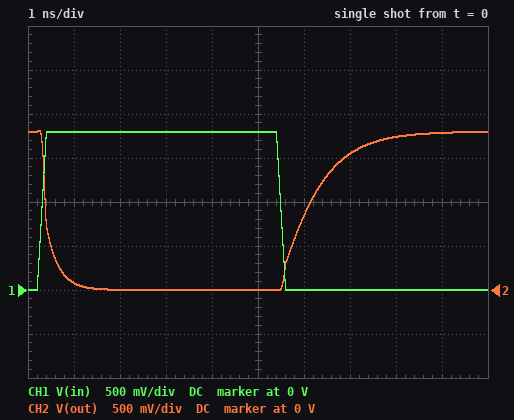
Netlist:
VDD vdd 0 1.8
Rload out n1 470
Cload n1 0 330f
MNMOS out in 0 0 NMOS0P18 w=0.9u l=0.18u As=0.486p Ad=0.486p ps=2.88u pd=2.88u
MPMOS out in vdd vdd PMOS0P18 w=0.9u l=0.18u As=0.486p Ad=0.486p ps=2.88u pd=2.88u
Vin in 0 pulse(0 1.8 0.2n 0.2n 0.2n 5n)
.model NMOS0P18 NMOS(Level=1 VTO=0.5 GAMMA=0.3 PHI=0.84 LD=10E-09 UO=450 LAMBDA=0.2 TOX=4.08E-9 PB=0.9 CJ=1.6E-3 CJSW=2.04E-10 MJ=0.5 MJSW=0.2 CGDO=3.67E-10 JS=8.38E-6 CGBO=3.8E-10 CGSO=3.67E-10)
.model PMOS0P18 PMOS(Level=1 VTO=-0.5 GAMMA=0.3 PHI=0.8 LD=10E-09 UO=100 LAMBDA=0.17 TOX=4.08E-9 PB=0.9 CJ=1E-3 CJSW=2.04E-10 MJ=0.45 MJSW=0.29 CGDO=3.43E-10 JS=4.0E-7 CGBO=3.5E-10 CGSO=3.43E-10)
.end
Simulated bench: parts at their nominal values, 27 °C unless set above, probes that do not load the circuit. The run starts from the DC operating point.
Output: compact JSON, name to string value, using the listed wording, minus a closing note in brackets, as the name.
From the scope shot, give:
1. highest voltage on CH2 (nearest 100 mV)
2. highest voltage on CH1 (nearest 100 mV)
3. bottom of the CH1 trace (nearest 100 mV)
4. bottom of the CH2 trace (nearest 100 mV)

{"highest voltage on CH2": "1.8 V", "highest voltage on CH1": "1.8 V", "bottom of the CH1 trace": "0 V", "bottom of the CH2 trace": "0 V"}
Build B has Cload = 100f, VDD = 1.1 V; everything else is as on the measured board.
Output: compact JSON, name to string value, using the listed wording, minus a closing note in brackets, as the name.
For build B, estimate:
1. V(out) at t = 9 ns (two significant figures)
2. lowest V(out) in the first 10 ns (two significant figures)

{"V(out) at t = 9 ns": "1.1 V", "lowest V(out) in the first 10 ns": "-12 mV"}
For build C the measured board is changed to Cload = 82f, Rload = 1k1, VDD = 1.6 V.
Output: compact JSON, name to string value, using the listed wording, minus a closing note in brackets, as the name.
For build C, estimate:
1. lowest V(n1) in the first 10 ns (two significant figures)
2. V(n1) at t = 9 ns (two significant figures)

{"lowest V(n1) in the first 10 ns": "-3.1 mV", "V(n1) at t = 9 ns": "1.6 V"}
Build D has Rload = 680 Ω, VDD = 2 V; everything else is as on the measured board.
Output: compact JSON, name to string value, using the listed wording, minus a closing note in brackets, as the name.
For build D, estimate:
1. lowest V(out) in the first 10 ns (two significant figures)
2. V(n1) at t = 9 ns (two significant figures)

{"lowest V(out) in the first 10 ns": "-3.3 mV", "V(n1) at t = 9 ns": "2.0 V"}
